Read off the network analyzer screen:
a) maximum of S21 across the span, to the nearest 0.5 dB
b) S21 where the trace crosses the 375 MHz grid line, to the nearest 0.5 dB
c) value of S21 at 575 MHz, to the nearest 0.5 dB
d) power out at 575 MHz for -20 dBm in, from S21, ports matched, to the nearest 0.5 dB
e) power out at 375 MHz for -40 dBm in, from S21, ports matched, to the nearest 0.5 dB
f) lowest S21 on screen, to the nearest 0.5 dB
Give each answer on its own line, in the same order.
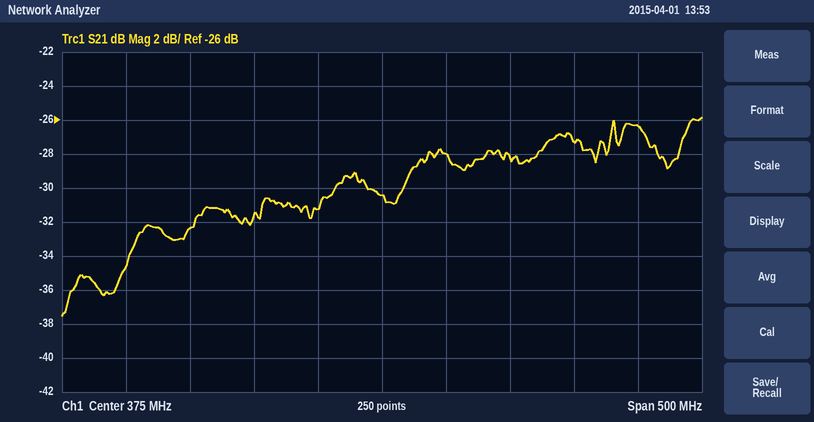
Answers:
-26.0 dB
-30.5 dB
-26.5 dB
-46.5 dBm
-70.5 dBm
-37.5 dB
